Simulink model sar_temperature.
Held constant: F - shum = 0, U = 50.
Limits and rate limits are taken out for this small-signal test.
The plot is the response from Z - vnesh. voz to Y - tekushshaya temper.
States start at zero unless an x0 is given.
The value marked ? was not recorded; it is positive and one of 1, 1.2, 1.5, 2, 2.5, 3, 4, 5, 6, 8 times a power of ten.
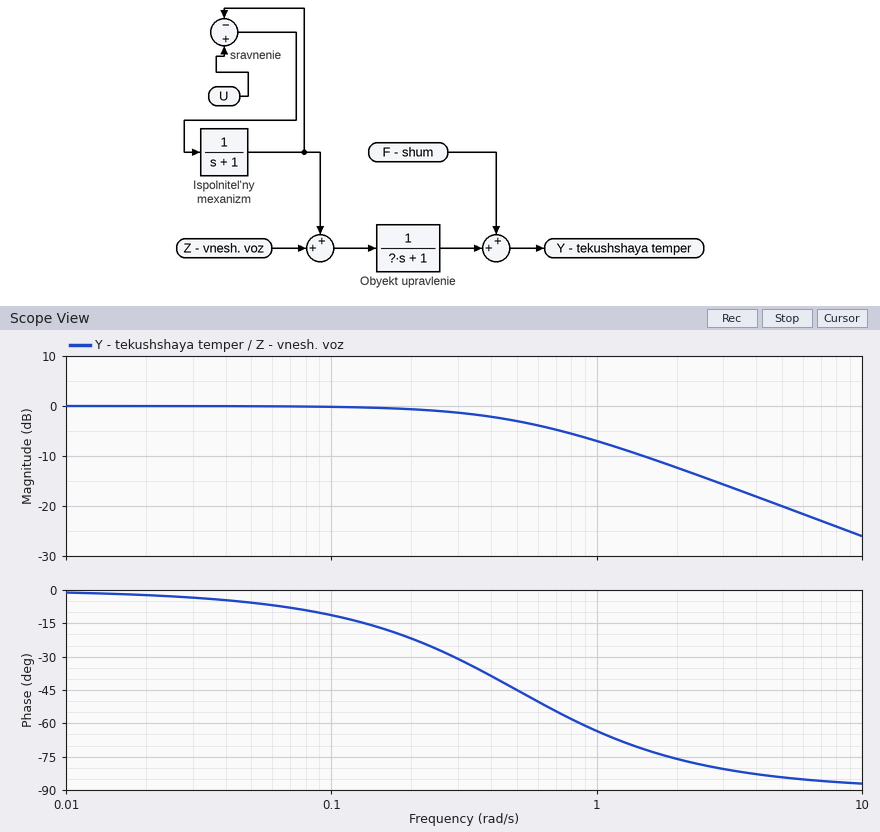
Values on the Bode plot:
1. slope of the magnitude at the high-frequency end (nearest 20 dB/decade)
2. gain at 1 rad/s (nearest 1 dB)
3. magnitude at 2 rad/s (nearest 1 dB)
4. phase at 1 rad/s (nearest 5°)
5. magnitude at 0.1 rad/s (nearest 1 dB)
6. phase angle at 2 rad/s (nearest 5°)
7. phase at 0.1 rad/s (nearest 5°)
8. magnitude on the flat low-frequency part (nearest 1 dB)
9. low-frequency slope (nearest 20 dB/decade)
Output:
-20 dB/decade
-7 dB
-12 dB
-65°
0 dB
-75°
-10°
0 dB
0 dB/decade
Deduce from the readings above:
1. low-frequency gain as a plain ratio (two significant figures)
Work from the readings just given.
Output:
1.0
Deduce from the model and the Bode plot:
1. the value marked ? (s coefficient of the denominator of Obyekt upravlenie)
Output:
2
